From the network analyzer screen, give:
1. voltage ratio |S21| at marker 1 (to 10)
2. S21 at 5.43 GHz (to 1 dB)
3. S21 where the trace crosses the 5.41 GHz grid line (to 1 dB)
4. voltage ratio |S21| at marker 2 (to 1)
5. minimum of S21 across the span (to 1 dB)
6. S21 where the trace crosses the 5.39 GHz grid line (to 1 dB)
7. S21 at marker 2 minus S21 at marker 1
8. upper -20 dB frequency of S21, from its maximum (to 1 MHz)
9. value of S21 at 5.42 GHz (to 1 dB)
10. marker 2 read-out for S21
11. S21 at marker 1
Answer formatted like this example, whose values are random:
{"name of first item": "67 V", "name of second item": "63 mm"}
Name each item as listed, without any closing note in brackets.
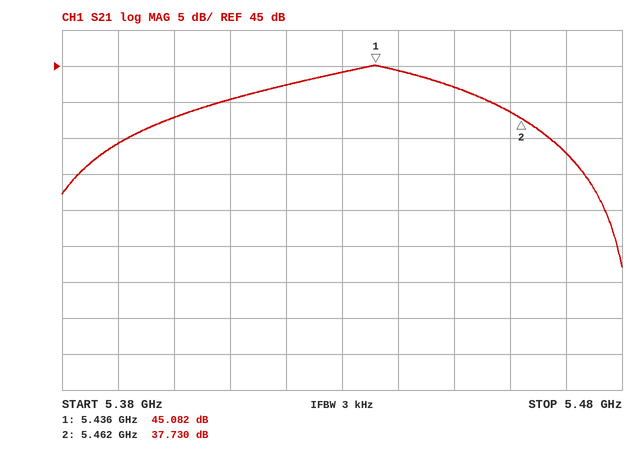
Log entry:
{"voltage ratio |S21| at marker 1": "180", "S21 at 5.43 GHz": "44 dB", "S21 where the trace crosses the 5.41 GHz grid line": "40 dB", "voltage ratio |S21| at marker 2": "77", "minimum of S21 across the span": "17 dB", "S21 where the trace crosses the 5.39 GHz grid line": "34 dB", "S21 at marker 2 minus S21 at marker 1": "-7.352 dB", "upper -20 dB frequency of S21, from its maximum": "5.477 GHz", "value of S21 at 5.42 GHz": "42 dB", "marker 2 read-out for S21": "37.730 dB", "S21 at marker 1": "45.082 dB"}
